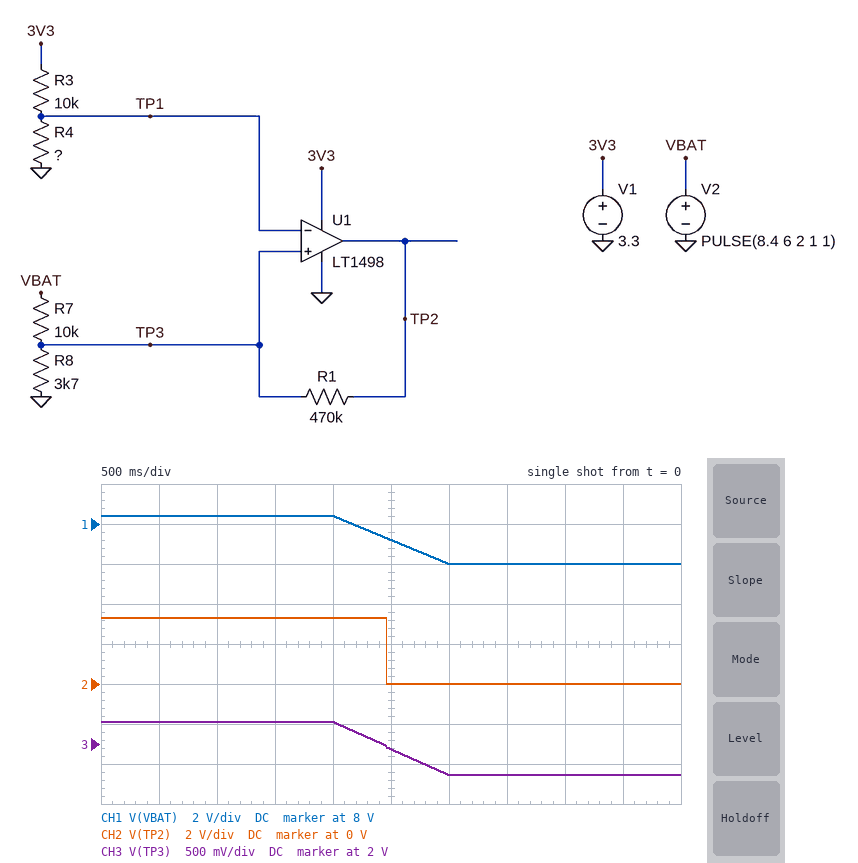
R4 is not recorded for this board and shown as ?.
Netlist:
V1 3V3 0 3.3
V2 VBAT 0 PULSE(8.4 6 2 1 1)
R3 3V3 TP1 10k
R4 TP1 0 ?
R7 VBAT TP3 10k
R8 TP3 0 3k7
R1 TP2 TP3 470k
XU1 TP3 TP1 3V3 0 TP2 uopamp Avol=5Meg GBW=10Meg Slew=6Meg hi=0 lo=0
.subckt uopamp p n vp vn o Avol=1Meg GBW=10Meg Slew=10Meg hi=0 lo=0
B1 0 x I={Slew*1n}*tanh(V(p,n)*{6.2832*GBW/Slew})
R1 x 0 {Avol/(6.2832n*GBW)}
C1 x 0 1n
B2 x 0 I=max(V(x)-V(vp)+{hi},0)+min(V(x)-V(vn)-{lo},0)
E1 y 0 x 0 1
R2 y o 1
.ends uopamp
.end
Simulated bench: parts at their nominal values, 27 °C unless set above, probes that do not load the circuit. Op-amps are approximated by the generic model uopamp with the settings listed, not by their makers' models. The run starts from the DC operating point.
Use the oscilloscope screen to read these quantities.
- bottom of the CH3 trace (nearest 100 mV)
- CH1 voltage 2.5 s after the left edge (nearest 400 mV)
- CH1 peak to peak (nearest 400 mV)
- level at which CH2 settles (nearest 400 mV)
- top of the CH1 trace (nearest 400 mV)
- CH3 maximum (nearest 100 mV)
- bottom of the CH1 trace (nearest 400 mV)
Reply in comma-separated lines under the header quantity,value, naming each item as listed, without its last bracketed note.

quantity,value
bottom of the CH3 trace,1.6 V
CH1 voltage 2.5 s after the left edge,7.2 V
CH1 peak to peak,2.4 V
level at which CH2 settles,0 V
top of the CH1 trace,8.4 V
CH3 maximum,2.3 V
bottom of the CH1 trace,6.0 V
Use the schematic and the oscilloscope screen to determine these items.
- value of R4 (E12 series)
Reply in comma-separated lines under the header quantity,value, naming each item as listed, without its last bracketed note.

quantity,value
value of R4,15 kΩ
